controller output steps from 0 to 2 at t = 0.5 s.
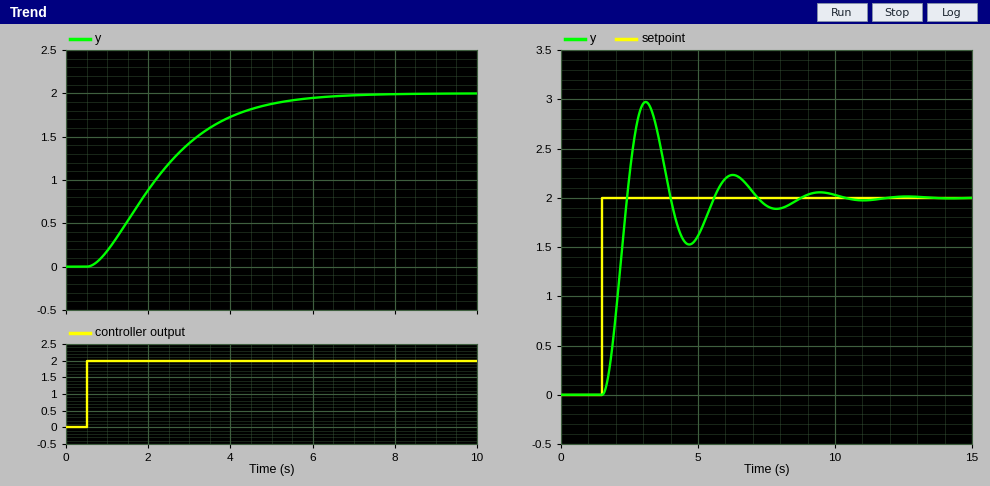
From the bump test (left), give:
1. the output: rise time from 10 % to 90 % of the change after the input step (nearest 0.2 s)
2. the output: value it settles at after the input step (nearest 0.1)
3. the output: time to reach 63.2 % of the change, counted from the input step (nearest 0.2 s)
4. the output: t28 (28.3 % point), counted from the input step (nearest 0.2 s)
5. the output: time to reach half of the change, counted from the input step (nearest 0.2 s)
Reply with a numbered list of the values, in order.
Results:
1. 3.4 s
2. 2.0
3. 2.2 s
4. 1.0 s
5. 1.6 s
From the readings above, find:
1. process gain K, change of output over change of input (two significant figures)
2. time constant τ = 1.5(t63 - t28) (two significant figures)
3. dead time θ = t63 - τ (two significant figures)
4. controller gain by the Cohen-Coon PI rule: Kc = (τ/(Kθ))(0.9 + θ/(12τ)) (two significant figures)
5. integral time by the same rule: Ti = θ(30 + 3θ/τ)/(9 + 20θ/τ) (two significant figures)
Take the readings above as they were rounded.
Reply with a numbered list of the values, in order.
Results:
1. 1.0
2. 1.8 s
3. 0.40 s
4. 4.1
5. 0.91 s
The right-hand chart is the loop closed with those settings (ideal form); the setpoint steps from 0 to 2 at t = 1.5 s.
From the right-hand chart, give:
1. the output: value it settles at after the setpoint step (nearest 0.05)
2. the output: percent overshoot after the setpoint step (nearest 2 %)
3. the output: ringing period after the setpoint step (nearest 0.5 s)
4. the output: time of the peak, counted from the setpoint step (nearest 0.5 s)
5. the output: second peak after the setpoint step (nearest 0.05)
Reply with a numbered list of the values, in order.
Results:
1. 2.00
2. 48 %
3. 3.0 s
4. 1.5 s
5. 2.25
